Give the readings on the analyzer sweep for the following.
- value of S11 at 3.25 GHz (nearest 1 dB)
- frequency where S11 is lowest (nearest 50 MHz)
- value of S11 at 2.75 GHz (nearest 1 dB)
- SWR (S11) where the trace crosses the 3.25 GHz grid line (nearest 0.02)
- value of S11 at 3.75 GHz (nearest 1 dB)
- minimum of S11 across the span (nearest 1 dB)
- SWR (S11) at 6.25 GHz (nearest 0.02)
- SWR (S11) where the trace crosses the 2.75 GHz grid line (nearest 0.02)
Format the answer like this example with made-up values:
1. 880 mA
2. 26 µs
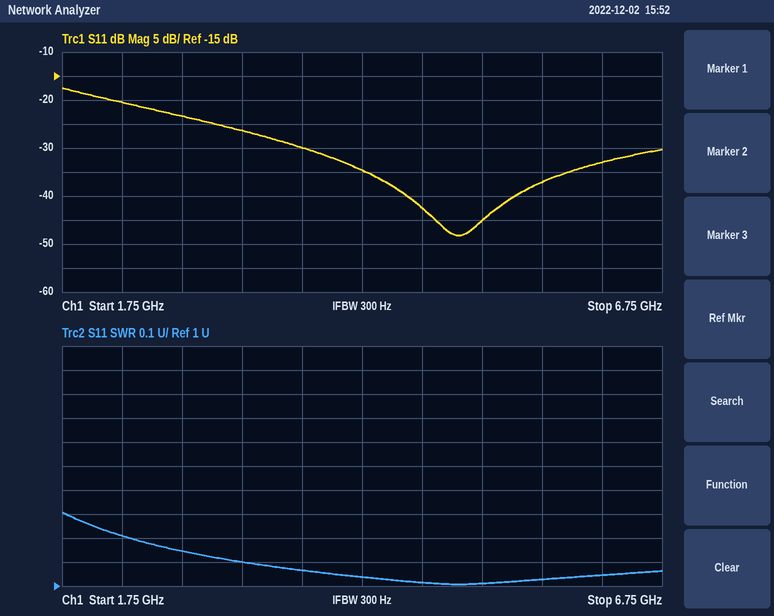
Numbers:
1. -26 dB
2. 5.05 GHz
3. -23 dB
4. 1.10
5. -30 dB
6. -48 dB
7. 1.04
8. 1.14
